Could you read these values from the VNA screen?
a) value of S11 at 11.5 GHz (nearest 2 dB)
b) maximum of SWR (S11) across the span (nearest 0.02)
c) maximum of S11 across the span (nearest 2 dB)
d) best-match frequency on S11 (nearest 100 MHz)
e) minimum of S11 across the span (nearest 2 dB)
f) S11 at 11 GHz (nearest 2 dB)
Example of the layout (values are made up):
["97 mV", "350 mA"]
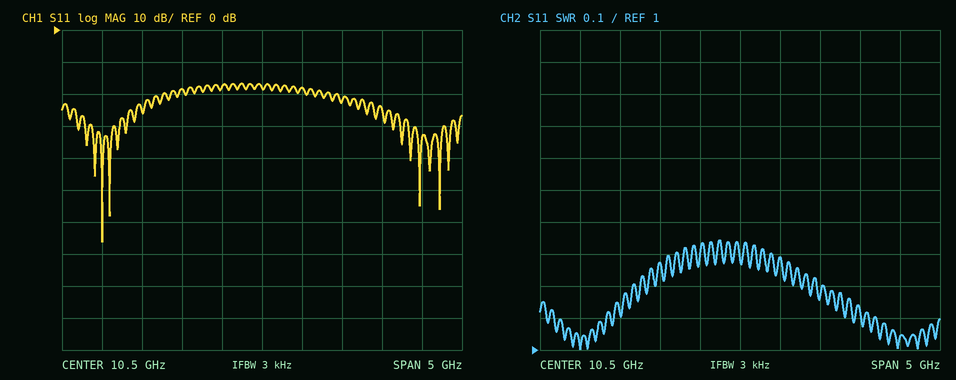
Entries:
["-22 dB", "1.34", "-16 dB", "8.5 GHz", "-66 dB", "-18 dB"]
